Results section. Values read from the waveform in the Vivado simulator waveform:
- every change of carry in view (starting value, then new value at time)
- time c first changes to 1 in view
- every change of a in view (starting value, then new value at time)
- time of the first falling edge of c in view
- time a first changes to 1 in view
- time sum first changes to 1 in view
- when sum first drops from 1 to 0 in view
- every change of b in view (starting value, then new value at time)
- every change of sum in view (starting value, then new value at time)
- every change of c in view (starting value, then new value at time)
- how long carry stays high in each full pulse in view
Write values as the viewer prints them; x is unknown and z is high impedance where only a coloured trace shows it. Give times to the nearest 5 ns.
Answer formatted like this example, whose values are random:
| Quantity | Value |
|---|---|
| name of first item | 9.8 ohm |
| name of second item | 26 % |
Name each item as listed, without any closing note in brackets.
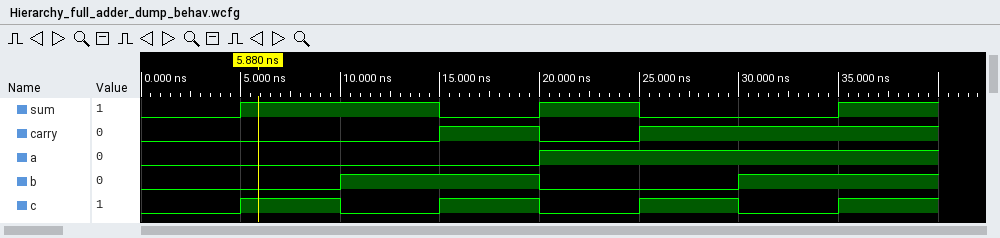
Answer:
| Quantity | Value |
|---|---|
| every change of carry in view | 0, 1 at 15 ns, 0 at 20 ns, 1 at 25 ns |
| time c first changes to 1 in view | 5 ns |
| every change of a in view | 0, 1 at 20 ns |
| time of the first falling edge of c in view | 10 ns |
| time a first changes to 1 in view | 20 ns |
| time sum first changes to 1 in view | 5 ns |
| when sum first drops from 1 to 0 in view | 15 ns |
| every change of b in view | 0, 1 at 10 ns, 0 at 20 ns, 1 at 30 ns |
| every change of sum in view | 0, 1 at 5 ns, 0 at 15 ns, 1 at 20 ns, 0 at 25 ns, 1 at 35 ns |
| every change of c in view | 0, 1 at 5 ns, 0 at 10 ns, 1 at 15 ns, 0 at 20 ns, 1 at 25 ns, 0 at 30 ns, 1 at 35 ns |
| how long carry stays high in each full pulse in view | 5 ns |
